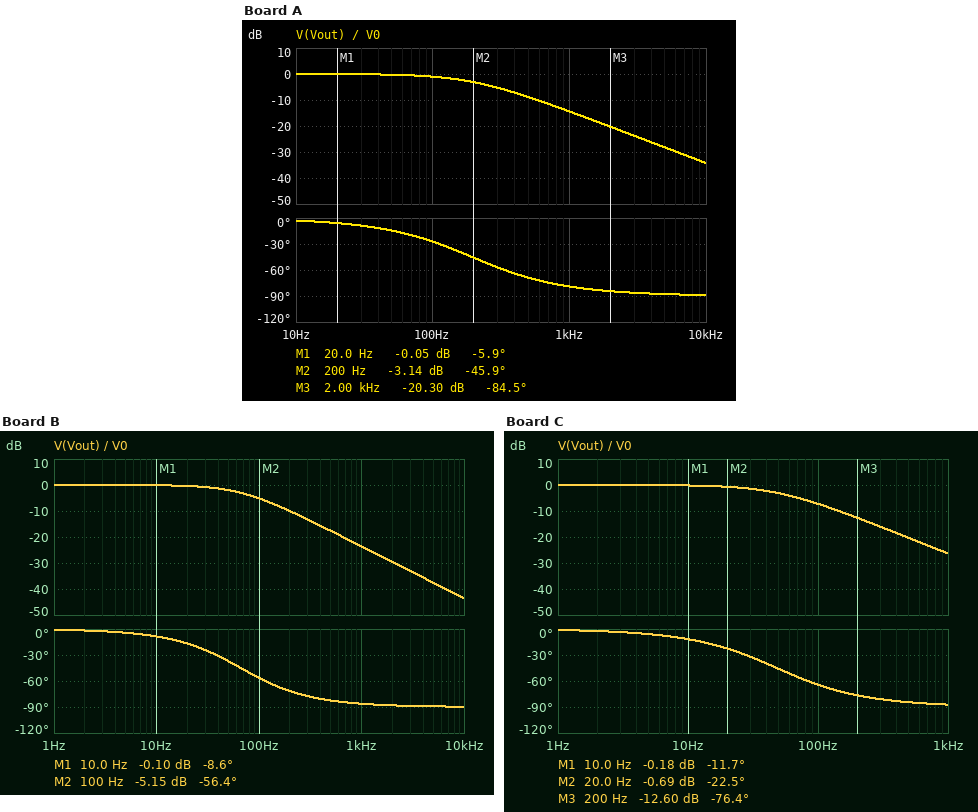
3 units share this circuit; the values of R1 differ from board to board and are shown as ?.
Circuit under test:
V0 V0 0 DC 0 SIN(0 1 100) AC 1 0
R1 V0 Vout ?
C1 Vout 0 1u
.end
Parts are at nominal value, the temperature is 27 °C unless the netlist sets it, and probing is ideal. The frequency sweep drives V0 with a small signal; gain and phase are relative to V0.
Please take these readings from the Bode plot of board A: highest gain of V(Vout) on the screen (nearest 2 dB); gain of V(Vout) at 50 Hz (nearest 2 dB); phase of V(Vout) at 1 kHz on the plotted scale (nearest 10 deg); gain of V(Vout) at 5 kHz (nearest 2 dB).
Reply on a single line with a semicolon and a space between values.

0 dB; 0 dB; -80 deg; -28 dB
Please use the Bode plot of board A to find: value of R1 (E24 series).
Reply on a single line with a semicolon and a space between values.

820 Ω
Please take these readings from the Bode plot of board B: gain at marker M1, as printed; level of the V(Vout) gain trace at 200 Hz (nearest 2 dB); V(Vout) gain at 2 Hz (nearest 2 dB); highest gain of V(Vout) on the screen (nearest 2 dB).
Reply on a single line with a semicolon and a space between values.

-0.10 dB; -10 dB; 0 dB; 0 dB
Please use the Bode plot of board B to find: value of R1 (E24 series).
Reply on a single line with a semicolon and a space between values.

2.4 kΩ
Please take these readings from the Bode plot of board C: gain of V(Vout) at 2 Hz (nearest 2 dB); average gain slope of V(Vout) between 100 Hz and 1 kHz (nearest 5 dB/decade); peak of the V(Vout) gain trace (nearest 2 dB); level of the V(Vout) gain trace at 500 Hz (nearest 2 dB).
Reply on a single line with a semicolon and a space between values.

0 dB; -20 dB/decade; 0 dB; -20 dB
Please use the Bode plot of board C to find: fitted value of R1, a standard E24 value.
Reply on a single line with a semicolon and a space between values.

3.3 kΩ
